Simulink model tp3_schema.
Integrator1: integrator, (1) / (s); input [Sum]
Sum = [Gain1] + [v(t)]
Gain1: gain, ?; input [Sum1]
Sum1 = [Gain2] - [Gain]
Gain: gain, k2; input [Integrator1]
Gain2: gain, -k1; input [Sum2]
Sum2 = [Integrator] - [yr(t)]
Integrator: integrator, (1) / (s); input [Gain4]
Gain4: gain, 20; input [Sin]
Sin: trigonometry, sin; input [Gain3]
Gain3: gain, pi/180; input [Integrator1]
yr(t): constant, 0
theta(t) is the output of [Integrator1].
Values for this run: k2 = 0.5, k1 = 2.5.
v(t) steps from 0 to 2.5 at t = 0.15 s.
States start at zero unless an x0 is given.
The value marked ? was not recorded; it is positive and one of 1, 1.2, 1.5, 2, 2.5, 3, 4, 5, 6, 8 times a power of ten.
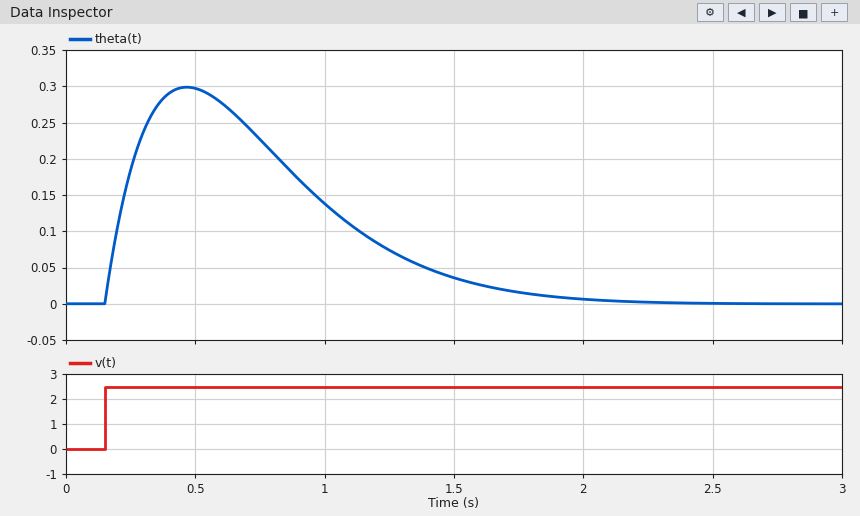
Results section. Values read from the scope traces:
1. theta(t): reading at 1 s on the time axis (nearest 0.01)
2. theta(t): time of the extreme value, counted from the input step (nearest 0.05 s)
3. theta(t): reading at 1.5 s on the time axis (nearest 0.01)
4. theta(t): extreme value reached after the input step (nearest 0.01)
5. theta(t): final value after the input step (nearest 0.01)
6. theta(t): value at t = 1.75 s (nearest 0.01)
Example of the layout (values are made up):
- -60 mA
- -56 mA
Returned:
- 0.14
- 0.30 s
- 0.04
- 0.30
- 0.00
- 0.02
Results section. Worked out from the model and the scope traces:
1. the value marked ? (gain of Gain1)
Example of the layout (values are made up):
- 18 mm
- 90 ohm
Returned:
- 12
